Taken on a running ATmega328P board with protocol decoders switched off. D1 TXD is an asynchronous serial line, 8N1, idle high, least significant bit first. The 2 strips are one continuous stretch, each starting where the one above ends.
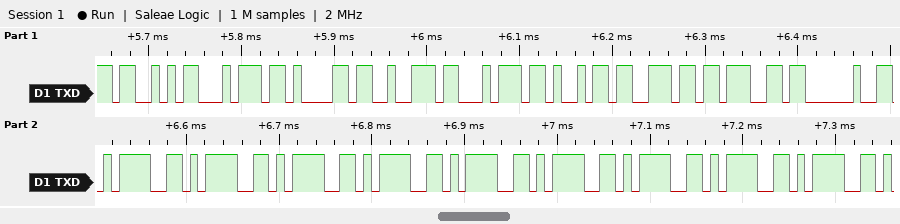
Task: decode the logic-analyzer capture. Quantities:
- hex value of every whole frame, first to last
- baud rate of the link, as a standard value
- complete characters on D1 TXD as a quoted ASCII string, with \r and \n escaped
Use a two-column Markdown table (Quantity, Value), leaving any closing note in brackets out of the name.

| Quantity | Value |
|---|---|
| hex value of every whole frame, first to last | 53 74 61 72 74 69 6E 67 20 3D 3D 3D 3D 3D 3D 3D 3D 3D |
| baud rate of the link, as a standard value | 115200 baud |
| complete characters on D1 TXD as a quoted ASCII string, with \r and \n escaped | "Starting =========" |
